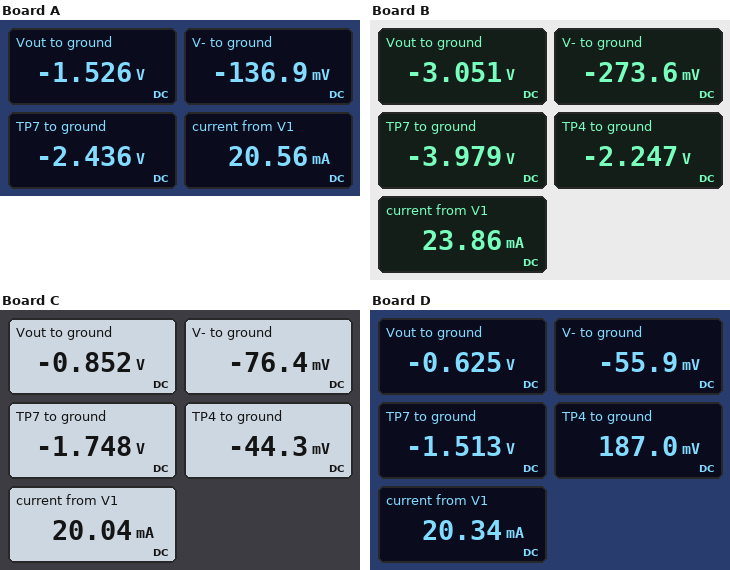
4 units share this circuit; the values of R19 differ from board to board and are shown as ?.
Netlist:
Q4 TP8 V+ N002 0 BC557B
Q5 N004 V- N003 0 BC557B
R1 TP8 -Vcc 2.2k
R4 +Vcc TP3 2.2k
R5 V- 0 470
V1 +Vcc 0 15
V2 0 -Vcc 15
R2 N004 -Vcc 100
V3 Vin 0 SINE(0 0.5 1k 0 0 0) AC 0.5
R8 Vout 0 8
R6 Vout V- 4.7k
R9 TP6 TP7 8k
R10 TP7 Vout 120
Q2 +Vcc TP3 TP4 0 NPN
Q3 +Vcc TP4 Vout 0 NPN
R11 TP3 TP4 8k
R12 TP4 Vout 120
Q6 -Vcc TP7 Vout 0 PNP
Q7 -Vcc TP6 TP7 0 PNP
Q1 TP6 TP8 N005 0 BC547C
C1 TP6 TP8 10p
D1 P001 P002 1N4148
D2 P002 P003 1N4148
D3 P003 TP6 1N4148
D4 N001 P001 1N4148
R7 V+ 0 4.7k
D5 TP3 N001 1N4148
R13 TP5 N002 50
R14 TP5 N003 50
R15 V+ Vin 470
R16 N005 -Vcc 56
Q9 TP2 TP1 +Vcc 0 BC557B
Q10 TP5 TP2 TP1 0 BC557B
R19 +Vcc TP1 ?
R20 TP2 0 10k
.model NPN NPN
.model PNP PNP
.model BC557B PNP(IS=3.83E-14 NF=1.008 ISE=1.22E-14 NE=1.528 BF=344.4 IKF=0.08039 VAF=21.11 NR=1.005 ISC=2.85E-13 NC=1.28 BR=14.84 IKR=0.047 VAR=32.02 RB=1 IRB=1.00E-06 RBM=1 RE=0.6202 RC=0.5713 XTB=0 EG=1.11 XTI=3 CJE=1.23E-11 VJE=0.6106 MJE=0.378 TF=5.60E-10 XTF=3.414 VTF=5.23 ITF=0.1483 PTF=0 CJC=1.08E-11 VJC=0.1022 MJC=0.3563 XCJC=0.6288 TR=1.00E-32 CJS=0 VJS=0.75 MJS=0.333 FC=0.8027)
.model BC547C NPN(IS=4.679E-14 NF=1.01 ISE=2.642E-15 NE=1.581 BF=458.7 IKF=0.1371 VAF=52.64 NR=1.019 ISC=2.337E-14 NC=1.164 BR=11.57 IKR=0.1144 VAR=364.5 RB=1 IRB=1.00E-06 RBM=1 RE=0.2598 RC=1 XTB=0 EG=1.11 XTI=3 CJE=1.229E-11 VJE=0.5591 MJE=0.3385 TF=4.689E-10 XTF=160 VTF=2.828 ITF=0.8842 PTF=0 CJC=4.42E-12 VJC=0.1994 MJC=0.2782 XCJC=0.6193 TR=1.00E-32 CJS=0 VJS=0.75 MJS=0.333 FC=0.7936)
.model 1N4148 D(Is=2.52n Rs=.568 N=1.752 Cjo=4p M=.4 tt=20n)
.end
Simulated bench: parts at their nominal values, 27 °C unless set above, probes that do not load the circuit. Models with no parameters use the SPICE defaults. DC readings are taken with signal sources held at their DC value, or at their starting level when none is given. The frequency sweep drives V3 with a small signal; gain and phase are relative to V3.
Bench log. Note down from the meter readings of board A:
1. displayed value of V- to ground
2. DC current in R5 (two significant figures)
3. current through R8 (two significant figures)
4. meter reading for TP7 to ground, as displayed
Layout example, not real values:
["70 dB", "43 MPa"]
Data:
["-136.9 mV", "290 µA", "190 mA", "-2.436 V"]
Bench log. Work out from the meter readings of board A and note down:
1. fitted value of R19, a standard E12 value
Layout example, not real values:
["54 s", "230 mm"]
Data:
["220 Ω"]
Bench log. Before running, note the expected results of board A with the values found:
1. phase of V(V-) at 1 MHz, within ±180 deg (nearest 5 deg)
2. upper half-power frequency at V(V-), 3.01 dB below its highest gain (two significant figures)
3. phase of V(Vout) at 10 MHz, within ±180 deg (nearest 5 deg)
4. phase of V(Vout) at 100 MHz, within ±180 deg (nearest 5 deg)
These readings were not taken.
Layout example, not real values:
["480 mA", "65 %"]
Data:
["-10 deg", "8.2 MHz", "-95 deg", "125 deg"]
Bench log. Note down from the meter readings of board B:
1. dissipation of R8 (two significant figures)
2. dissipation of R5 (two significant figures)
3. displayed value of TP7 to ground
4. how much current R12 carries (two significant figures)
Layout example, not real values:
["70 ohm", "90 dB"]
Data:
["1.2 W", "160 µW", "-3.979 V", "6.7 mA"]
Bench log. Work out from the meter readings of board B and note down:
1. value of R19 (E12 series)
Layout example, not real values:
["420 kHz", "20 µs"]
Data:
["120 Ω"]
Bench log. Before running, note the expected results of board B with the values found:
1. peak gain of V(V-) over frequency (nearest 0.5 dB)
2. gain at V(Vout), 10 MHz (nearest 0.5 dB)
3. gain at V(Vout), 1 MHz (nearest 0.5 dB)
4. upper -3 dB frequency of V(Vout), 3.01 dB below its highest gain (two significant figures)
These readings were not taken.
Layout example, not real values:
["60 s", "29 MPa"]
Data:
["-1.0 dB", "17.5 dB", "20.0 dB", "11 MHz"]
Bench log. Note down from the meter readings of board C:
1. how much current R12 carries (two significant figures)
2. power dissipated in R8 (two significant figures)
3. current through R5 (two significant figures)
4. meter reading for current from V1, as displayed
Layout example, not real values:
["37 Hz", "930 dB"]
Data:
["6.7 mA", "91 mW", "160 µA", "20.04 mA"]
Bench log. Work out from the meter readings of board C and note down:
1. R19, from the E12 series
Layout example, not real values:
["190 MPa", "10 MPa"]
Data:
["330 Ω"]
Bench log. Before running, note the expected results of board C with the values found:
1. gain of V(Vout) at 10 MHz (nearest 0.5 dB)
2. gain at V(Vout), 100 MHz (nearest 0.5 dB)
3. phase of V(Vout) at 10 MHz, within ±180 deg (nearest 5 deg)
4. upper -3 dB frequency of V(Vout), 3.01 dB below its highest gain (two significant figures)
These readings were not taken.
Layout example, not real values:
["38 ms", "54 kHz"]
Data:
["16.5 dB", "-16.5 dB", "-100 deg", "9.9 MHz"]
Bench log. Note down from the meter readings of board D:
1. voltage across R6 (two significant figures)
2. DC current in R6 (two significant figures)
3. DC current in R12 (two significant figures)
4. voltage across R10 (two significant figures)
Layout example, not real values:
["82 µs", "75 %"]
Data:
["570 mV", "120 µA", "6.8 mA", "890 mV"]
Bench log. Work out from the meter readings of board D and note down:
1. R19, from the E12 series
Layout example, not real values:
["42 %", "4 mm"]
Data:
["390 Ω"]
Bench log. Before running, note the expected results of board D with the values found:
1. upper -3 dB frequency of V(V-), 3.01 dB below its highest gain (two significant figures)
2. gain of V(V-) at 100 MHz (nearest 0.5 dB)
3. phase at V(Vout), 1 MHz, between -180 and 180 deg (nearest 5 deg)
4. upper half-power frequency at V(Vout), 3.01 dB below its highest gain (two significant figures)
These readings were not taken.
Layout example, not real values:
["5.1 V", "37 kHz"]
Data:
["7.1 MHz", "-10.0 dB", "-10 deg", "9.5 MHz"]
